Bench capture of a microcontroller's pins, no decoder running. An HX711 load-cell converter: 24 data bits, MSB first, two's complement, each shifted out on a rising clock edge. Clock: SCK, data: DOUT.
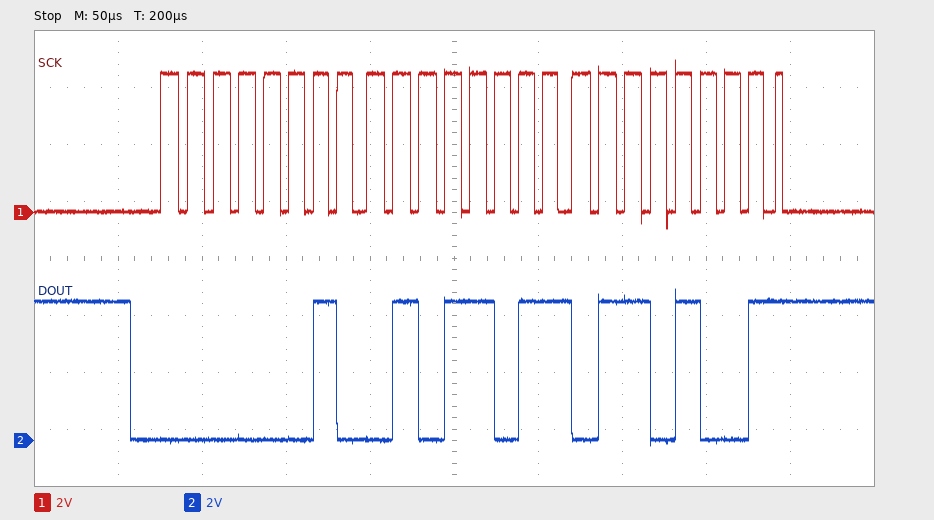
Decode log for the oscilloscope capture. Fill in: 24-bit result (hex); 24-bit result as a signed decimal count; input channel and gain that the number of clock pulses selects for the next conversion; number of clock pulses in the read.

0x025B69
154473
channel A, gain 128
25
